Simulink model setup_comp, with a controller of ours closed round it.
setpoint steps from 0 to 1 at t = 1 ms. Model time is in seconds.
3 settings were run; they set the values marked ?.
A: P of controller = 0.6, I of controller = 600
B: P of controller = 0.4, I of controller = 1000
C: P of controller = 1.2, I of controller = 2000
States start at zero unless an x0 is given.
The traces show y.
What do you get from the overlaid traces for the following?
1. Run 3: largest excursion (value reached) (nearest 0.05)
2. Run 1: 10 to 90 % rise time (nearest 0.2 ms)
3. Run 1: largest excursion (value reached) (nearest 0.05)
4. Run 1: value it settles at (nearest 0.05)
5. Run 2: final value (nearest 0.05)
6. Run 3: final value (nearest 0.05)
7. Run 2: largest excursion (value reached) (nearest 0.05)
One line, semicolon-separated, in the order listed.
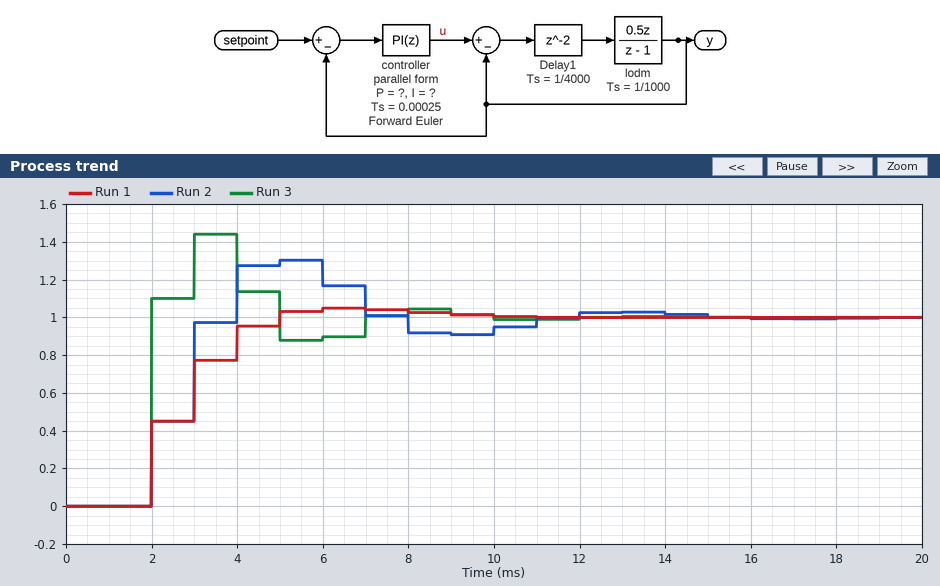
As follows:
1.45; 2.0 ms; 1.05; 1.00; 1.00; 1.00; 1.30
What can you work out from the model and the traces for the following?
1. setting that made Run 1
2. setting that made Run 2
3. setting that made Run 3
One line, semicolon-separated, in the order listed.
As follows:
A; B; C
